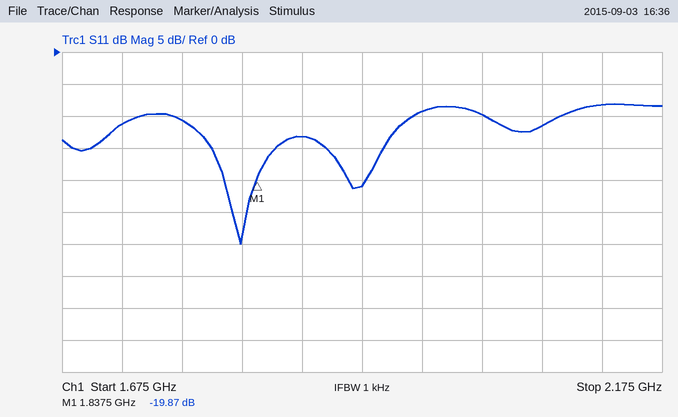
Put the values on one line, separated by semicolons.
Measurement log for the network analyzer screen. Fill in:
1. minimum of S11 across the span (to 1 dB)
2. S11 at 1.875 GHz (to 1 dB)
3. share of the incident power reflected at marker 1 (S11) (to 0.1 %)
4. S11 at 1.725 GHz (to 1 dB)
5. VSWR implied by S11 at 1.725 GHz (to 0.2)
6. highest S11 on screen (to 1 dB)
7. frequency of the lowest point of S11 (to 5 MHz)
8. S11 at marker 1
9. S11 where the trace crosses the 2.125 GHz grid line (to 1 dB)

-30 dB; -13 dB; 1.0 %; -11 dB; 1.8; -8 dB; 1.825 GHz; -19.87 dB; -8 dB
